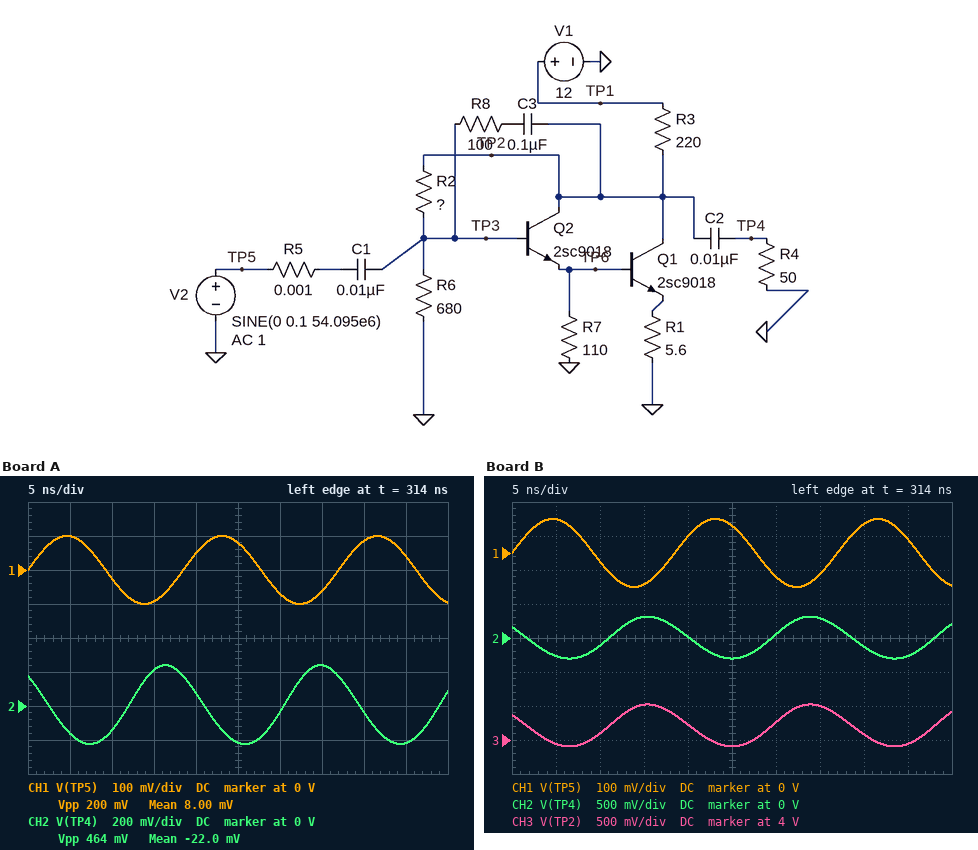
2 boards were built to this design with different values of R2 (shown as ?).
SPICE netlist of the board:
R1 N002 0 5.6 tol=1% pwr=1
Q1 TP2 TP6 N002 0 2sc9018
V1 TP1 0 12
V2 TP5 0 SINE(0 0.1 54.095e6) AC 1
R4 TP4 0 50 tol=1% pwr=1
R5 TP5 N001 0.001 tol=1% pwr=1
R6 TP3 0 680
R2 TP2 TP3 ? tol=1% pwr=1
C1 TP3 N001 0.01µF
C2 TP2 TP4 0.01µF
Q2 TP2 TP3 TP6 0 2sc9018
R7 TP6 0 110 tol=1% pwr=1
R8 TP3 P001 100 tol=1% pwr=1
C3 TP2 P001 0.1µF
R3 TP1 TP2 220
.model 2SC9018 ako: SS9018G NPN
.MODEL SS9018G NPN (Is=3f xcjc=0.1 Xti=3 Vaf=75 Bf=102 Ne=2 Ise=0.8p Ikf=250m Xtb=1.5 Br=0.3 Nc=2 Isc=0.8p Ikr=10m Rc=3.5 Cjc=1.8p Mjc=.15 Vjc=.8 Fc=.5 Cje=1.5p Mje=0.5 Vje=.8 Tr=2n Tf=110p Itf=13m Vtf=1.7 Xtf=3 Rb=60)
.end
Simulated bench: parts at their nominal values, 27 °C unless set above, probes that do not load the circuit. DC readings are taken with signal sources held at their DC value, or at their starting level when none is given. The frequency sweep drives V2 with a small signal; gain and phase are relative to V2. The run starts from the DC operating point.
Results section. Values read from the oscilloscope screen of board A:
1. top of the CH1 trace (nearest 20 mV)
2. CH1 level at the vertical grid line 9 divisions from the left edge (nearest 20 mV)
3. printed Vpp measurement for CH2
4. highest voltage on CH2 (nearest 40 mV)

100 mV
40 mV
464 mV
240 mV
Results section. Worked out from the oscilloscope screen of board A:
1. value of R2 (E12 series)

220 Ω
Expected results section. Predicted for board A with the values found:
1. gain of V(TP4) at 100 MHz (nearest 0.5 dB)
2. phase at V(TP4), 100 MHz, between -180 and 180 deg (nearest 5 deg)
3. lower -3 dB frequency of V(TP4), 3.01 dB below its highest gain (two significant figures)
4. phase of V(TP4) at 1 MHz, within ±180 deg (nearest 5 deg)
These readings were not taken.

4.0 dB
105 deg
930 kHz
-125 deg
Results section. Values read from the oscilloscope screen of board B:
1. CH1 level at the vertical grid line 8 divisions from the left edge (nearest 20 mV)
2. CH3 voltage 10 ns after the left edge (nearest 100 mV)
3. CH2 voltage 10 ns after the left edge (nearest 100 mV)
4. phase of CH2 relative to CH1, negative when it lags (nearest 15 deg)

80 mV
4.1 V
-100 mV
150 deg
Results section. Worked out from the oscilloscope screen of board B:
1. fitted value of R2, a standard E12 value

1 kΩ
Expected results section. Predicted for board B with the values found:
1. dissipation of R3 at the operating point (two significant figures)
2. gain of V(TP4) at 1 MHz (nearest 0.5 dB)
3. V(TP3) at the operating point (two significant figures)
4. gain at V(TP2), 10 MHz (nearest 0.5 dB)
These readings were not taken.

280 mW
9.0 dB
1.7 V
11.0 dB
